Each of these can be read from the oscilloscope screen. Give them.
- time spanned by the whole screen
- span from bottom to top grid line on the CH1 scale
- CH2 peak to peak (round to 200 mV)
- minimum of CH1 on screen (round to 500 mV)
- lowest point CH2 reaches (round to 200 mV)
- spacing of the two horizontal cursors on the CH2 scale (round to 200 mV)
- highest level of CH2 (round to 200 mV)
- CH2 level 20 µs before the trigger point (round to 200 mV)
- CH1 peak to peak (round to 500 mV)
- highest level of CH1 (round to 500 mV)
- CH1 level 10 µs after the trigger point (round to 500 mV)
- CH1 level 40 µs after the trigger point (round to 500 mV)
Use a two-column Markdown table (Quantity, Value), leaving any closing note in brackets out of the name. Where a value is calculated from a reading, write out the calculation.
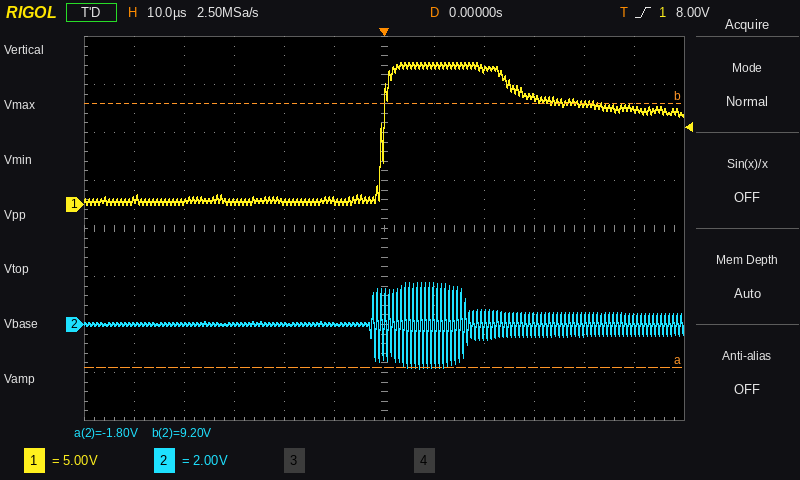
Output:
| Quantity | Value |
|---|---|
| time spanned by the whole screen | 120 µs |
| span from bottom to top grid line on the CH1 scale | 40 V |
| CH2 peak to peak | 1.8 V − (-1.8 V) = 3.6 V |
| minimum of CH1 on screen | 0.0 V |
| lowest point CH2 reaches | -1.8 V |
| spacing of the two horizontal cursors on the CH2 scale | 11.0 V |
| highest level of CH2 | 1.8 V |
| CH2 level 20 µs before the trigger point | 0.0 V |
| CH1 peak to peak | 15.0 V − (0.0 V) = 15.0 V |
| highest level of CH1 | 15.0 V |
| CH1 level 10 µs after the trigger point | 14.5 V |
| CH1 level 40 µs after the trigger point | 10.5 V |
